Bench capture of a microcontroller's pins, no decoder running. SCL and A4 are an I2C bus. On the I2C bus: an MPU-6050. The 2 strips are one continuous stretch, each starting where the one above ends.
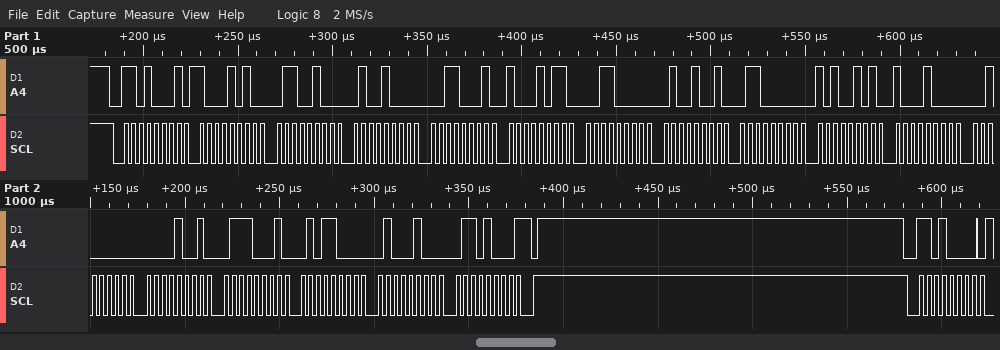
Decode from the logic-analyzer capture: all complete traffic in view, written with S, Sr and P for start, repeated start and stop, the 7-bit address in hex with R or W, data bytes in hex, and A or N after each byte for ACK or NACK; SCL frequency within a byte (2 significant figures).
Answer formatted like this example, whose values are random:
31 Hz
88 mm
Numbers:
S 68R A 8A A 64 A 48 A 31 A 8B A 30 A 49 A 60 A A5 A 88 A 20 A 09 A 71 A 58 A 44 A 68 N P S 68W A
250 kHz
